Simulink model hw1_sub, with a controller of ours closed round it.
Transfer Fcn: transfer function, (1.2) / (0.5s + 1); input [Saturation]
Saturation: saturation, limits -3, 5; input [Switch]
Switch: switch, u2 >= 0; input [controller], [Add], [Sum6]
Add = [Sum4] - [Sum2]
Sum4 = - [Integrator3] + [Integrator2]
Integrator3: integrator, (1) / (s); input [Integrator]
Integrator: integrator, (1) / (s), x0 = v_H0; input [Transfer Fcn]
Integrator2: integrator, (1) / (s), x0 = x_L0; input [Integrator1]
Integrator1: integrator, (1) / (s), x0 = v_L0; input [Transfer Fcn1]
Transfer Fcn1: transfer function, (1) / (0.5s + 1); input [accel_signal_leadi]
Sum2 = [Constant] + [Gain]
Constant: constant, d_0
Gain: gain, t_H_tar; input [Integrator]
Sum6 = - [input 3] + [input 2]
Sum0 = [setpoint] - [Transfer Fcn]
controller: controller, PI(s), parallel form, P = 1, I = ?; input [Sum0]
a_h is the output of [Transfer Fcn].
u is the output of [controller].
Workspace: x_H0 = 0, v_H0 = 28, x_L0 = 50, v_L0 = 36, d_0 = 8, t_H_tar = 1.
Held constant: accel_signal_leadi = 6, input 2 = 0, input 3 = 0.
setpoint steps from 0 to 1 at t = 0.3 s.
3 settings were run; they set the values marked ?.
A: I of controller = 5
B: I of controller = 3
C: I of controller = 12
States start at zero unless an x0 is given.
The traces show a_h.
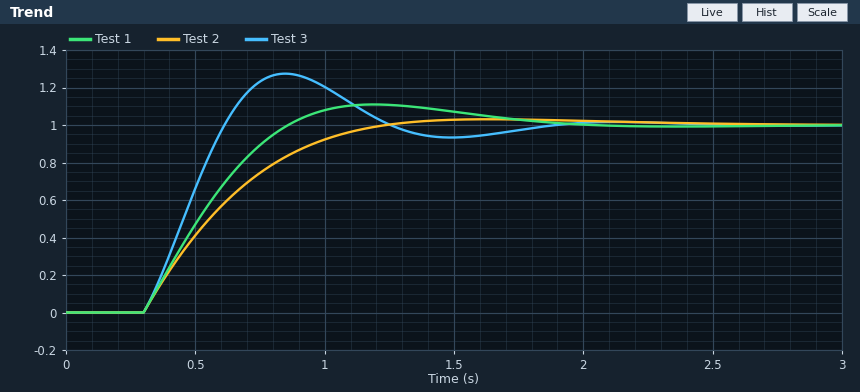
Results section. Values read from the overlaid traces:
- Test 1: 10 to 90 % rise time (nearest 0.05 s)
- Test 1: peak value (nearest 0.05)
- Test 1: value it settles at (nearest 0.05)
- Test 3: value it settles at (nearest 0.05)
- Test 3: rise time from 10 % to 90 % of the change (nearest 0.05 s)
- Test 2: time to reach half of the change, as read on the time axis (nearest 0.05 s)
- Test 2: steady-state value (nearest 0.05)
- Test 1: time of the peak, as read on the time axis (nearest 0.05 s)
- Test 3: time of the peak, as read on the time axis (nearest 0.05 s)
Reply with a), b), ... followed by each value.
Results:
a) 0.40 s
b) 1.10
c) 1.00
d) 1.00
e) 0.25 s
f) 0.55 s
g) 1.00
h) 1.20 s
i) 0.85 s
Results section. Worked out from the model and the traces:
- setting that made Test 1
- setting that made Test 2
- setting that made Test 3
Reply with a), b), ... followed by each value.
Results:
a) A
b) B
c) C
